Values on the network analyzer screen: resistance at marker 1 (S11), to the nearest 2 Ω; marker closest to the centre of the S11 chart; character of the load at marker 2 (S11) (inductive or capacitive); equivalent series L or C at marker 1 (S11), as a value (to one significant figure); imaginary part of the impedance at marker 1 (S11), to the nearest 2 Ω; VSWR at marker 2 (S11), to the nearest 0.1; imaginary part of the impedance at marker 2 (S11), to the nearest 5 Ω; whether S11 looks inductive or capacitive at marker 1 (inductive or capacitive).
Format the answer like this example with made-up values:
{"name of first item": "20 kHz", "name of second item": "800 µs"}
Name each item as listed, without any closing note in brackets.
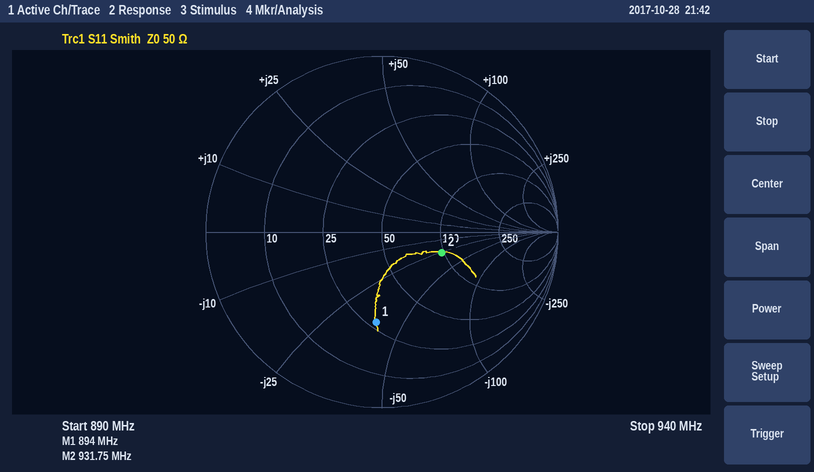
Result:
{"resistance at marker 1 (S11), to the nearest 2 Ω": "28 Ω", "marker closest to the centre of the S11 chart": "marker 2", "character of the load at marker 2 (S11)": "capacitive", "equivalent series L or C at marker 1 (S11), as a value": "5 pF", "imaginary part of the impedance at marker 1 (S11), to the nearest 2 Ω": "-38 Ω", "VSWR at marker 2 (S11), to the nearest 0.1": "2.1", "imaginary part of the impedance at marker 2 (S11), to the nearest 5 Ω": "-25 Ω", "whether S11 looks inductive or capacitive at marker 1": "capacitive"}
